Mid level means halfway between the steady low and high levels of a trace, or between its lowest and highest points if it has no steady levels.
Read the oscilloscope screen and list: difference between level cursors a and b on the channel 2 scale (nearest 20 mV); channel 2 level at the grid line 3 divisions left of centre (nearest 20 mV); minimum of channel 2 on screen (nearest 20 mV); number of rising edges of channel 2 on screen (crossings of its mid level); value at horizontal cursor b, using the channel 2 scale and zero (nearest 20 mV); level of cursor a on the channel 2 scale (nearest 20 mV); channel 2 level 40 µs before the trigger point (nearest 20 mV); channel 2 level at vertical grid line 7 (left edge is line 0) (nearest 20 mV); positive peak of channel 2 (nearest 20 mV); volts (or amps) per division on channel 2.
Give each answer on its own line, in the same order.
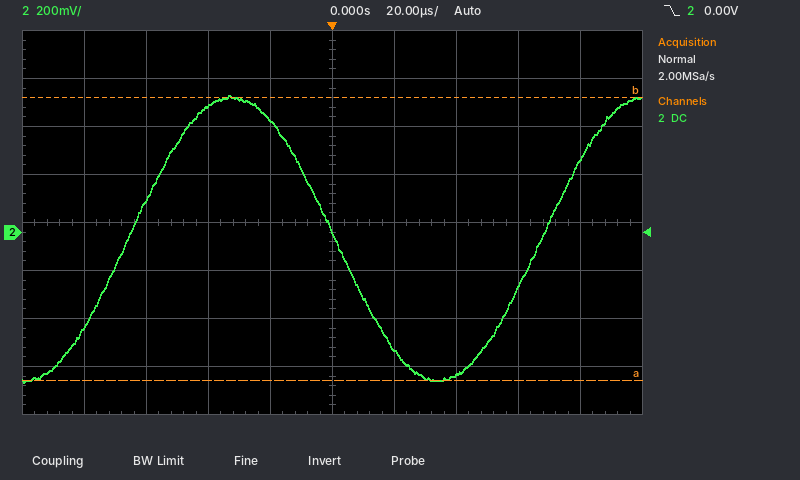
1.18 V
140 mV
-620 mV
2
560 mV
-620 mV
520 mV
-600 mV
560 mV
200 mV
